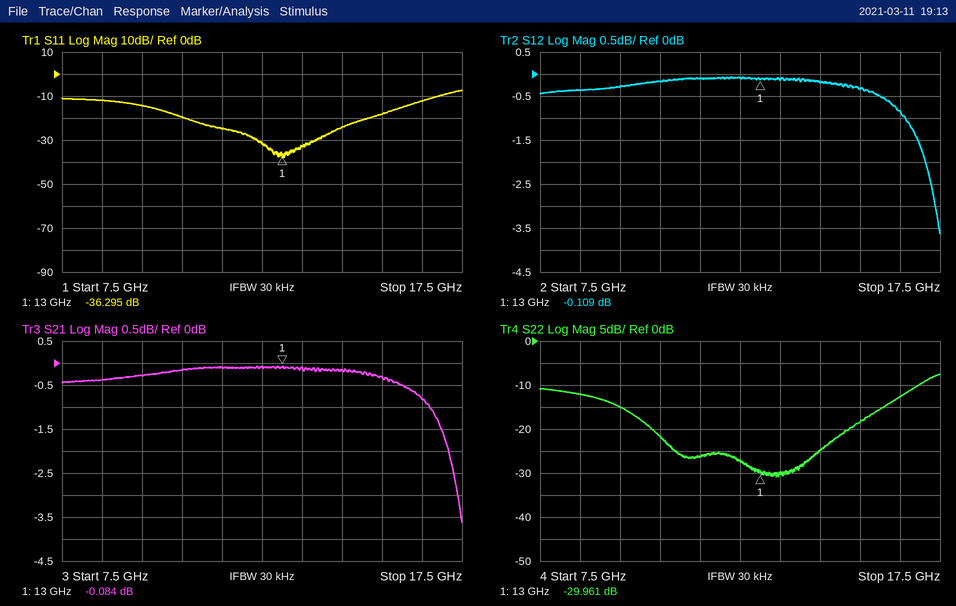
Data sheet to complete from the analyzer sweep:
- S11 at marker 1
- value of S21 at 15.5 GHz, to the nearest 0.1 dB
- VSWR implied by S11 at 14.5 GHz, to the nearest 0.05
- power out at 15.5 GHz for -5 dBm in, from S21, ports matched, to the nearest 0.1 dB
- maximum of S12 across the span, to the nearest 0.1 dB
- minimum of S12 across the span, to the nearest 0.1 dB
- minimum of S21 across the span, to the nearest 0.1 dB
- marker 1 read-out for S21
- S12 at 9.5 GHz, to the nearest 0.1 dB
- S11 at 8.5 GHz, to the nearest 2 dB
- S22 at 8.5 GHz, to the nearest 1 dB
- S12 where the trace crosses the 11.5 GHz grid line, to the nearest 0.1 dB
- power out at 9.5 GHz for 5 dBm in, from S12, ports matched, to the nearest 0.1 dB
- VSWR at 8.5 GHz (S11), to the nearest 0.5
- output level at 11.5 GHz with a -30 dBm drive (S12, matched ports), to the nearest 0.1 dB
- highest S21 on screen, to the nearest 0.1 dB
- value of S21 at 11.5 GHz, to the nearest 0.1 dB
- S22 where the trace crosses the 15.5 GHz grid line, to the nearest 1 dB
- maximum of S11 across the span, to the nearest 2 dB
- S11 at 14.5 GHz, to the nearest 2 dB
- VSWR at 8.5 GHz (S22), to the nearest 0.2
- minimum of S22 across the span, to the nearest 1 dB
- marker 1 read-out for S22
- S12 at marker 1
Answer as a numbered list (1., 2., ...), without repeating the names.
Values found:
1. -36.295 dB
2. -0.3 dB
3. 1.15
4. -5.3 dBm
5. -0.1 dB
6. -3.6 dB
7. -3.6 dB
8. -0.084 dB
9. -0.3 dB
10. -12 dB
11. -12 dB
12. -0.1 dB
13. 4.7 dBm
14. 1.5
15. -30.1 dBm
16. -0.1 dB
17. -0.1 dB
18. -18 dB
19. -8 dB
20. -24 dB
21. 1.6
22. -31 dB
23. -29.961 dB
24. -0.109 dB
